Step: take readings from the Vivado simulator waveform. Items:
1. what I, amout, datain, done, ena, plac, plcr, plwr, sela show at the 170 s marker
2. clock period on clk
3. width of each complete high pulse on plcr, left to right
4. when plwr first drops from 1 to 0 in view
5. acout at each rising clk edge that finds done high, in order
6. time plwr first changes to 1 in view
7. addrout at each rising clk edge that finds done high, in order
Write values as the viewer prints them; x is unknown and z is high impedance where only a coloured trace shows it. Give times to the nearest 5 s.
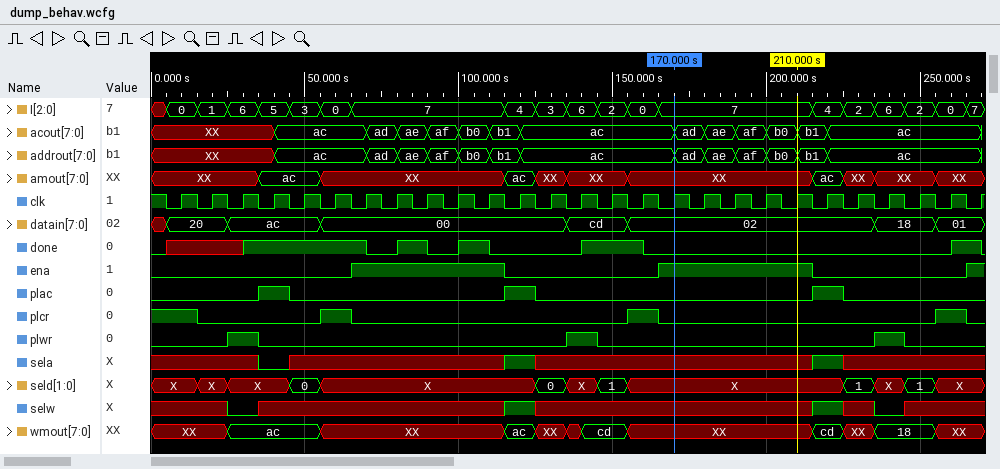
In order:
I=7, amout=XX, datain=02, done=0, ena=1, plac=0, plcr=0, plwr=0, sela=x
10 s
10 s, 10 s, 10 s
35 s
XX, ac, ac, ac, ae, b0, ac, ac, ac
25 s
XX, ac, ac, ac, ae, b0, ac, ac, ac
